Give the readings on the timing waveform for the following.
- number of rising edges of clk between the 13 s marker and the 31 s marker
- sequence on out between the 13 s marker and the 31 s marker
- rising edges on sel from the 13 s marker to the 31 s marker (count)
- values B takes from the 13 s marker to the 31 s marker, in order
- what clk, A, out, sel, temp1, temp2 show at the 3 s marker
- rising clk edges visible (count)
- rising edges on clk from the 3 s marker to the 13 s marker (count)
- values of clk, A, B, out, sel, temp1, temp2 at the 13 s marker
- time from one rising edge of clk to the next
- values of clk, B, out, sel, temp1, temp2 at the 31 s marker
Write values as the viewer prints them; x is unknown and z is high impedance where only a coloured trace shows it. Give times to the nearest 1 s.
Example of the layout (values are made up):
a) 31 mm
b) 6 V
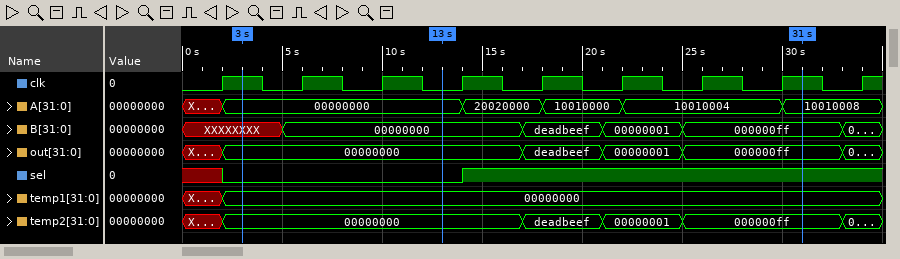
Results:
a) 5
b) 00000000, deadbeef, 00000001, 000000ff
c) 1
d) 00000000, deadbeef, 00000001, 000000ff
e) clk=1, A=00000000, out=00000000, sel=0, temp1=00000000, temp2=00000000
f) 9
g) 2
h) clk=0, A=00000000, B=00000000, out=00000000, sel=0, temp1=00000000, temp2=00000000
i) 4 s
j) clk=1, B=000000ff, out=000000ff, sel=1, temp1=00000000, temp2=000000ff
